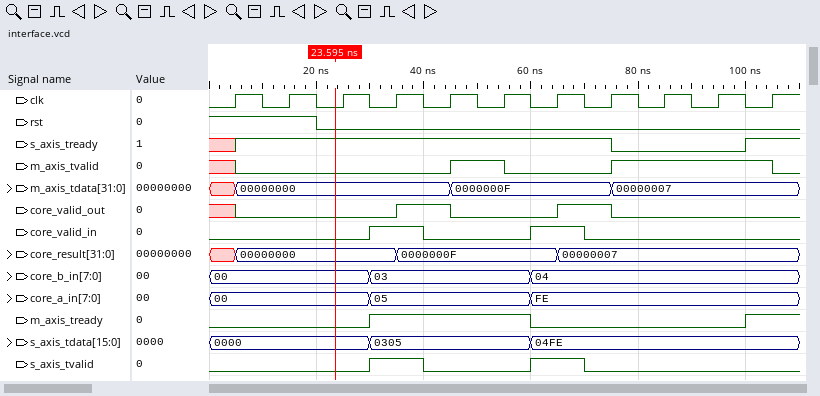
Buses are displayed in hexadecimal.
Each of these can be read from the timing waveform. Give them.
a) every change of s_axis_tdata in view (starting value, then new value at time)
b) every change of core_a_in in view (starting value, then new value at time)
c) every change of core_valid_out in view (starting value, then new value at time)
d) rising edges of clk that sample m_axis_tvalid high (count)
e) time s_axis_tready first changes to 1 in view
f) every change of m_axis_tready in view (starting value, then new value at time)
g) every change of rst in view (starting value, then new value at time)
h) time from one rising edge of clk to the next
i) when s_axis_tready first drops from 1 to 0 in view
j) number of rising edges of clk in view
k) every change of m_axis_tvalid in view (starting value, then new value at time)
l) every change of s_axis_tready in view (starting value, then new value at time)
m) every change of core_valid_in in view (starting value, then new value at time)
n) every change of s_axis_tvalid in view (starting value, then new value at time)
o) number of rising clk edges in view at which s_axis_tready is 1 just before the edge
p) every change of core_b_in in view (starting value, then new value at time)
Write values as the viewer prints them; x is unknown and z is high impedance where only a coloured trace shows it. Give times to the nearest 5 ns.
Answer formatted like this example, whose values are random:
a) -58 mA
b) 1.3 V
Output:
a) 0000, 0305 at 30 ns, 04FE at 60 ns
b) 00, 05 at 30 ns, FE at 60 ns
c) x, 0 at 5 ns, 1 at 35 ns, 0 at 45 ns, 1 at 65 ns, 0 at 75 ns
d) 4
e) 5 ns
f) 0, 1 at 30 ns, 0 at 60 ns, 1 at 100 ns
g) 1, 0 at 20 ns
h) 10 ns
i) 75 ns
j) 11
k) x, 0 at 5 ns, 1 at 45 ns, 0 at 55 ns, 1 at 75 ns, 0 at 105 ns
l) x, 1 at 5 ns, 0 at 75 ns, 1 at 100 ns
m) 0, 1 at 30 ns, 0 at 40 ns, 1 at 60 ns, 0 at 70 ns
n) 0, 1 at 30 ns, 0 at 40 ns, 1 at 60 ns, 0 at 70 ns
o) 8
p) 00, 03 at 30 ns, 04 at 60 ns
